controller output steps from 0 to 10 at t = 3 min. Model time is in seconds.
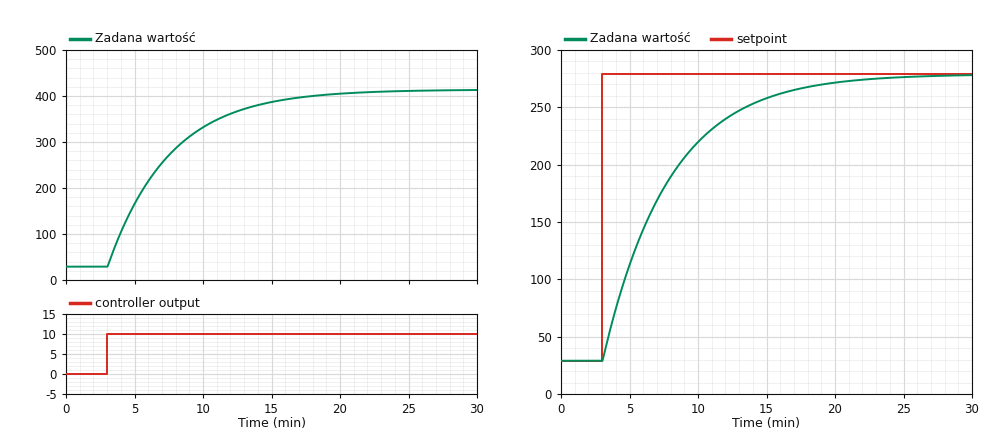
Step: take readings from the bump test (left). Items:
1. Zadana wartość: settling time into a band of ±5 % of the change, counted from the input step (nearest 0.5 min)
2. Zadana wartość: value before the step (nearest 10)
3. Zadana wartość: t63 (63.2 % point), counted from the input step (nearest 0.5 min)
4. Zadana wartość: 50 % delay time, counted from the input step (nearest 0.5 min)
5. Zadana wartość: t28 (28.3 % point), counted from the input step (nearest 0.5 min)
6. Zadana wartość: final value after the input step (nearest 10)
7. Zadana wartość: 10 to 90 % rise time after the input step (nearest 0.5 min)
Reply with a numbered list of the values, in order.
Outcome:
1. 13.5 min
2. 30
3. 4.5 min
4. 3.0 min
5. 1.5 min
6. 410
7. 10.0 min
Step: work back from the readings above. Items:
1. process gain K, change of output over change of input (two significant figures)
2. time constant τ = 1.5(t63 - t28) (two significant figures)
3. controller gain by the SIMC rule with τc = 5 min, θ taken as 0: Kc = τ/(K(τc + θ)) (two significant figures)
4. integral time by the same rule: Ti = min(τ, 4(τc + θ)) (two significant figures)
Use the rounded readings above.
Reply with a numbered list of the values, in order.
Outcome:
1. 38
2. 4.5 min
3. 0.024
4. 4.5 min
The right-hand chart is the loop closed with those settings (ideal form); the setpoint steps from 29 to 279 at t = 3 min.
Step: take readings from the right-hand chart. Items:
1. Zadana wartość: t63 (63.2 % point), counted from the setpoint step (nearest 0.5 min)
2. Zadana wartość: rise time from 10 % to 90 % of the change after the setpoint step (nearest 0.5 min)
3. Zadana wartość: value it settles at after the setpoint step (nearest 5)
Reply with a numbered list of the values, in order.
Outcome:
1. 5.0 min
2. 10.5 min
3. 280
